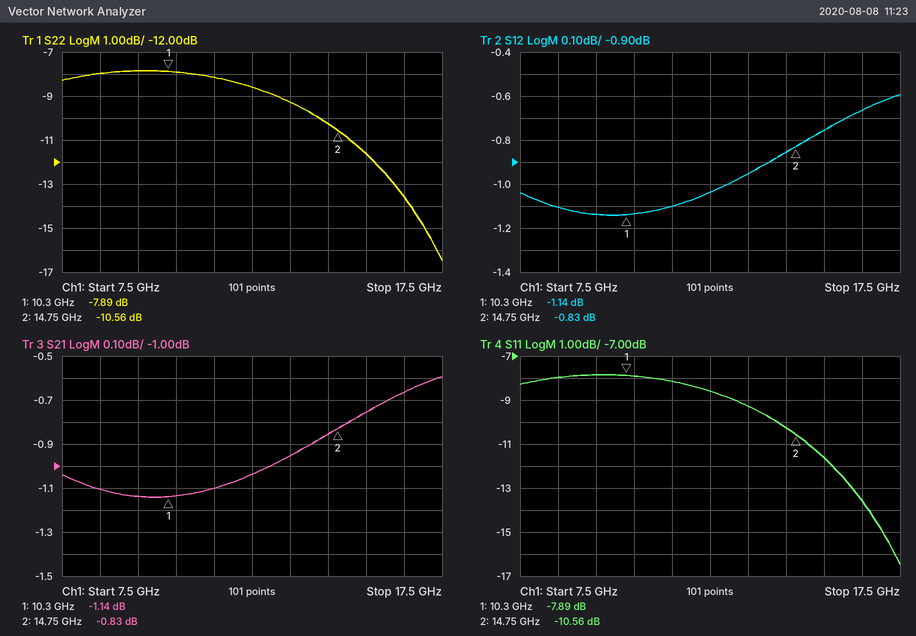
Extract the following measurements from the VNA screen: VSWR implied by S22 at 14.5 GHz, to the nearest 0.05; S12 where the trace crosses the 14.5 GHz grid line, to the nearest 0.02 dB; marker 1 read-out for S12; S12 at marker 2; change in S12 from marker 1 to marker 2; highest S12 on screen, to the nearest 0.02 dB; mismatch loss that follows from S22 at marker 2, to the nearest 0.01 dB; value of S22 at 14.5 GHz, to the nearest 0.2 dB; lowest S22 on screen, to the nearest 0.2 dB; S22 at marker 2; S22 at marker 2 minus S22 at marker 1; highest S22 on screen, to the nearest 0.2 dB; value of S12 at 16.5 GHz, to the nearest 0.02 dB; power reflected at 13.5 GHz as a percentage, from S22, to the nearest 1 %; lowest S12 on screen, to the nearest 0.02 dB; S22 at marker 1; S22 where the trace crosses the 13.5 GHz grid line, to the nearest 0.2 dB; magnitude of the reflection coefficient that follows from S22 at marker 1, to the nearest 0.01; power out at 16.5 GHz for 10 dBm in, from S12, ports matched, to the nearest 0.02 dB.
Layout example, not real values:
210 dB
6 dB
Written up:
1.90
-0.86 dB
-1.14 dB
-0.83 dB
0.31 dB
-0.60 dB
0.40 dB
-10.2 dB
-16.4 dB
-10.56 dB
-2.67 dB
-7.8 dB
-0.66 dB
12 %
-1.14 dB
-7.89 dB
-9.2 dB
0.40
9.34 dBm
